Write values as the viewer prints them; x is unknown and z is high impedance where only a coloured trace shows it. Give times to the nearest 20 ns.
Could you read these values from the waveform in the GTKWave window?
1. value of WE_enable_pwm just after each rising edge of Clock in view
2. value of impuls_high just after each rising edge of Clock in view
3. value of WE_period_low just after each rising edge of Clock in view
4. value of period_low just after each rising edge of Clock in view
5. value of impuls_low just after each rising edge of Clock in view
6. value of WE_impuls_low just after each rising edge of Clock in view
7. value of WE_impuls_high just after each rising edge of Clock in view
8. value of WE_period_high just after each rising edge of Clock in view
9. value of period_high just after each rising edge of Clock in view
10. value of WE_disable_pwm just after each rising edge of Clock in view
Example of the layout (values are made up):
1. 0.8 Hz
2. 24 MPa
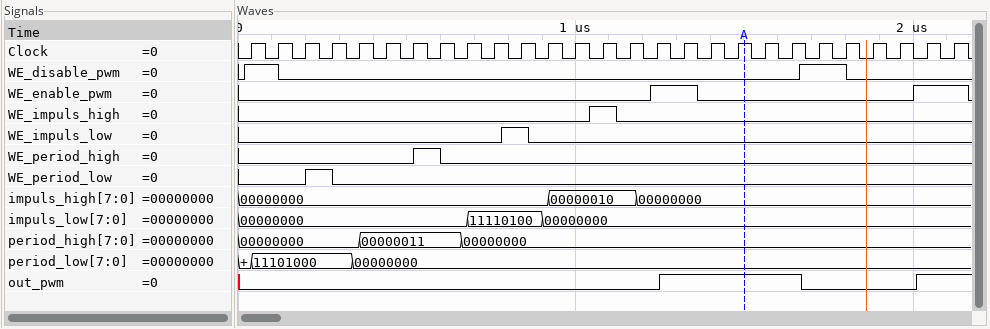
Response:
1. 0 0 0 0 0 0 0 0 0 0 0 0 0 0 0 1 1 0 0 0 0 0 0 0 0 1 1
2. 00000000, 00000000, 00000000, 00000000, 00000000, 00000000, 00000000, 00000000, 00000000, 00000000, 00000000, 00000010, 00000010, 00000010, 00000010, 00000000, 00000000, 00000000, 00000000, 00000000, 00000000, 00000000, 00000000, 00000000, 00000000, 00000000, 00000000
3. 0 0 1 0 0 0 0 0 0 0 0 0 0 0 0 0 0 0 0 0 0 0 0 0 0 0 0
4. 11101000, 11101000, 11101000, 11101000, 00000000, 00000000, 00000000, 00000000, 00000000, 00000000, 00000000, 00000000, 00000000, 00000000, 00000000, 00000000, 00000000, 00000000, 00000000, 00000000, 00000000, 00000000, 00000000, 00000000, 00000000, 00000000, 00000000
5. 00000000, 00000000, 00000000, 00000000, 00000000, 00000000, 00000000, 00000000, 11110100, 11110100, 11110100, 00000000, 00000000, 00000000, 00000000, 00000000, 00000000, 00000000, 00000000, 00000000, 00000000, 00000000, 00000000, 00000000, 00000000, 00000000, 00000000
6. 0 0 0 0 0 0 0 0 0 0 1 0 0 0 0 0 0 0 0 0 0 0 0 0 0 0 0
7. 0 0 0 0 0 0 0 0 0 0 0 0 0 1 0 0 0 0 0 0 0 0 0 0 0 0 0
8. 0 0 0 0 0 0 1 0 0 0 0 0 0 0 0 0 0 0 0 0 0 0 0 0 0 0 0
9. 00000000, 00000000, 00000000, 00000000, 00000011, 00000011, 00000011, 00000011, 00000000, 00000000, 00000000, 00000000, 00000000, 00000000, 00000000, 00000000, 00000000, 00000000, 00000000, 00000000, 00000000, 00000000, 00000000, 00000000, 00000000, 00000000, 00000000
10. 1 0 0 0 0 0 0 0 0 0 0 0 0 0 0 0 0 0 0 0 0 1 0 0 0 0 0
